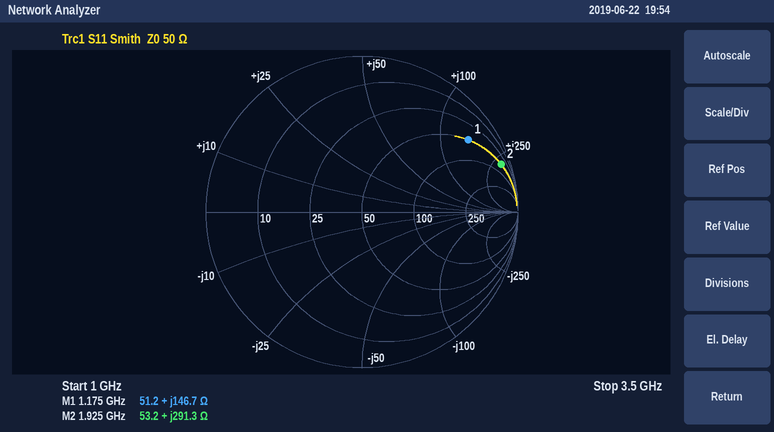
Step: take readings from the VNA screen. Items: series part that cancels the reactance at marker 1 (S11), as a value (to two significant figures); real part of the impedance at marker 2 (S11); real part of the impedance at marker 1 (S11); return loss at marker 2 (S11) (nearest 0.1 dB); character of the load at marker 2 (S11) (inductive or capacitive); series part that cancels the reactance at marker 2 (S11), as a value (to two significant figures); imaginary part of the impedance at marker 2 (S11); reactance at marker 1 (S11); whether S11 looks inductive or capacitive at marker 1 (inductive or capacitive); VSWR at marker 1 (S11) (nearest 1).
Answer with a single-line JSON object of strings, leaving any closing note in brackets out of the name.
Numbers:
{"series part that cancels the reactance at marker 1 (S11), as a value": "920 fF", "real part of the impedance at marker 2": "53.2 Ω", "real part of the impedance at marker 1": "51.2 Ω", "return loss at marker 2 (S11)": "0.5 dB", "character of the load at marker 2 (S11)": "inductive", "series part that cancels the reactance at marker 2 (S11), as a value": "280 fF", "imaginary part of the impedance at marker 2": "+291.3 Ω", "reactance at marker 1": "+146.7 Ω", "whether S11 looks inductive or capacitive at marker 1": "inductive", "VSWR at marker 1 (S11)": "10"}
